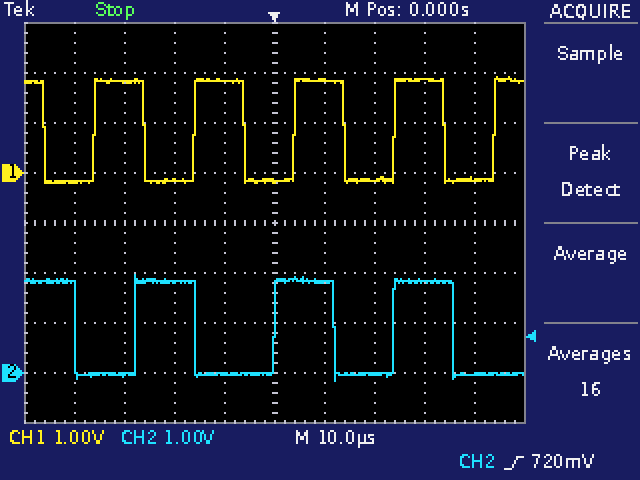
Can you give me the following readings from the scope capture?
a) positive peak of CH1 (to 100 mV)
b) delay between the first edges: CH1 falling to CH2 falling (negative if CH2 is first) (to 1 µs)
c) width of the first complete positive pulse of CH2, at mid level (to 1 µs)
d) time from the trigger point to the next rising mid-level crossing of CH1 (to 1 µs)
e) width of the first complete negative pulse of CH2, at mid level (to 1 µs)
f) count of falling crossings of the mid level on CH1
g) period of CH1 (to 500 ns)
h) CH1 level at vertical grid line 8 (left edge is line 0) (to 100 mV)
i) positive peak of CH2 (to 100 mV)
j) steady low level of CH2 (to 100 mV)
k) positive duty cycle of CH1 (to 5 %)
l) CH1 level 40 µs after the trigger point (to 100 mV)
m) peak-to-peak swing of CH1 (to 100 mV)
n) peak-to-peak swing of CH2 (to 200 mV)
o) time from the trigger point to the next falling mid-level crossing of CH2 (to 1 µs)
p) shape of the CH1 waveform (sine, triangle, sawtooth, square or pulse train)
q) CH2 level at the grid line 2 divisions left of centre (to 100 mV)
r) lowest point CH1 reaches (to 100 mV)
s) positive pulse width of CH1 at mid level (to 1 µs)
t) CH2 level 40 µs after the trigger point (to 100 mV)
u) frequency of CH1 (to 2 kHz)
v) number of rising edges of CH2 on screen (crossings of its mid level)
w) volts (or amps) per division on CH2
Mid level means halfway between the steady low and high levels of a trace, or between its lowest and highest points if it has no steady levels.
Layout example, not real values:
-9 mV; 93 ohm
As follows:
1.9 V; +6 µs; 12 µs; 4 µs; 12 µs; 5; 20.0 µs; 1.9 V; 2.0 V; 0.0 V; 50 %; -100 mV; 2.1 V; 2.2 V; 12 µs; square; 1.8 V; -200 mV; 10 µs; 0.0 V; 50 kHz; 3; 1 V
